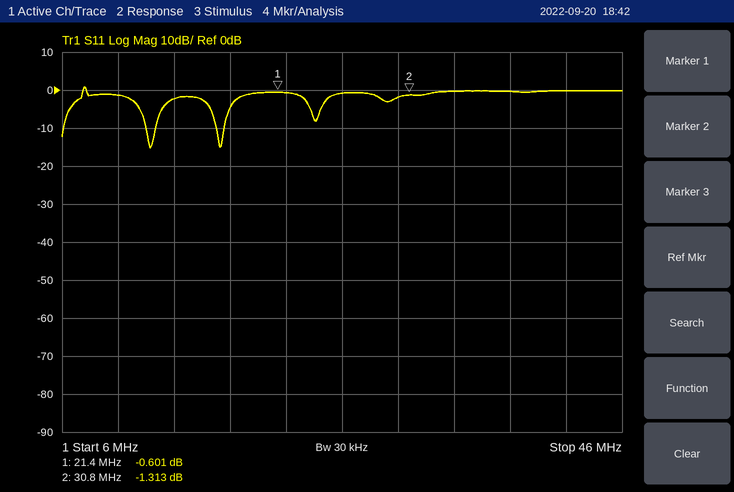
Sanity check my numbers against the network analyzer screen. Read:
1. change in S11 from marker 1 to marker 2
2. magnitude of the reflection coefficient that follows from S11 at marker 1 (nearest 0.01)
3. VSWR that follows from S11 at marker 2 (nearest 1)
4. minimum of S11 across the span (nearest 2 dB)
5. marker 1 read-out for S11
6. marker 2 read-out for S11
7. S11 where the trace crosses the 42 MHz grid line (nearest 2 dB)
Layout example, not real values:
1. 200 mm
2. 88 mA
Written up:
1. -0.712 dB
2. 0.93
3. 13
4. -16 dB
5. -0.601 dB
6. -1.313 dB
7. 0 dB
